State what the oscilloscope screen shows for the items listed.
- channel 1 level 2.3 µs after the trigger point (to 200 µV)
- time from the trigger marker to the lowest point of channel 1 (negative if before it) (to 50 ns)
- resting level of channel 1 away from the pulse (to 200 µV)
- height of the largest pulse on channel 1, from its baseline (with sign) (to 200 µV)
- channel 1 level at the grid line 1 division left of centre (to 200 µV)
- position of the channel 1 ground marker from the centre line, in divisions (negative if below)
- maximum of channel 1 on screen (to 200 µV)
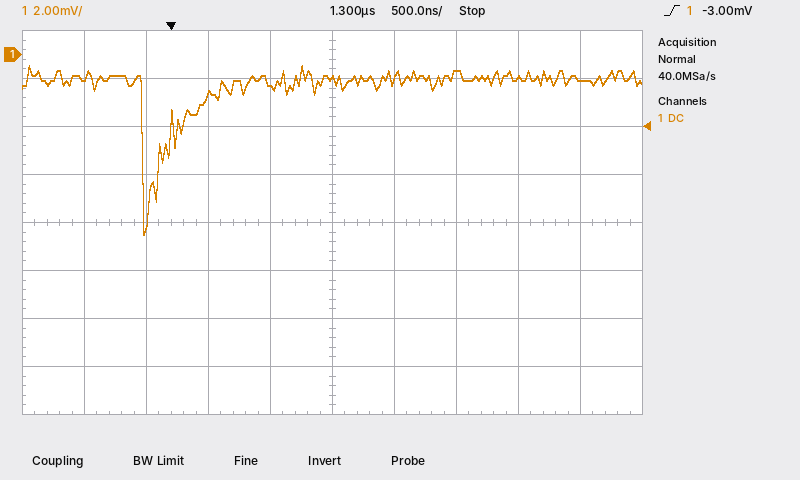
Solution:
-800 µV
-200 ns
-1.0 mV
-6.4 mV
-1.2 mV
+3.5 div
-400 µV
